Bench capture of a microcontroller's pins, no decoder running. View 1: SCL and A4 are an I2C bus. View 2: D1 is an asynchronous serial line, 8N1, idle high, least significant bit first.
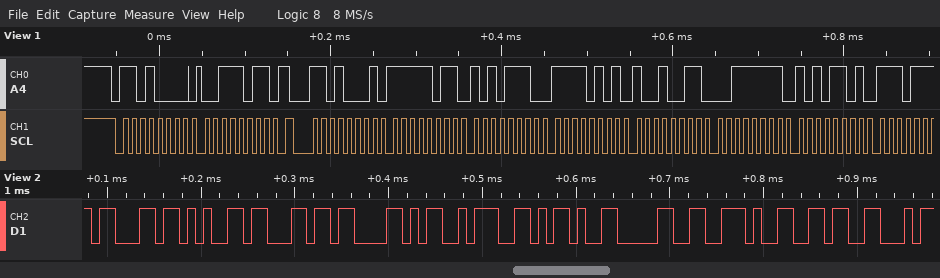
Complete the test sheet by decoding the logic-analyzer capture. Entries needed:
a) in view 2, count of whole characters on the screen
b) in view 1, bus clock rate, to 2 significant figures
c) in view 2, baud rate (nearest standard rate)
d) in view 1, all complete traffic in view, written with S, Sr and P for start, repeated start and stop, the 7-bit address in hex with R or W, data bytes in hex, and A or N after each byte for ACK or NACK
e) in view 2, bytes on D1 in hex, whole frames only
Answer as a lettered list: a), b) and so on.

a) 9
b) 100 kHz
c) 115200 baud
d) S 68W A 3B A Sr 68R A FB A AE A F5 A 93 A 3F A AD A
e) 0x63 0x65 0x6C 0x58 0x3A 0x2D 0x30 0x2E 0x36
